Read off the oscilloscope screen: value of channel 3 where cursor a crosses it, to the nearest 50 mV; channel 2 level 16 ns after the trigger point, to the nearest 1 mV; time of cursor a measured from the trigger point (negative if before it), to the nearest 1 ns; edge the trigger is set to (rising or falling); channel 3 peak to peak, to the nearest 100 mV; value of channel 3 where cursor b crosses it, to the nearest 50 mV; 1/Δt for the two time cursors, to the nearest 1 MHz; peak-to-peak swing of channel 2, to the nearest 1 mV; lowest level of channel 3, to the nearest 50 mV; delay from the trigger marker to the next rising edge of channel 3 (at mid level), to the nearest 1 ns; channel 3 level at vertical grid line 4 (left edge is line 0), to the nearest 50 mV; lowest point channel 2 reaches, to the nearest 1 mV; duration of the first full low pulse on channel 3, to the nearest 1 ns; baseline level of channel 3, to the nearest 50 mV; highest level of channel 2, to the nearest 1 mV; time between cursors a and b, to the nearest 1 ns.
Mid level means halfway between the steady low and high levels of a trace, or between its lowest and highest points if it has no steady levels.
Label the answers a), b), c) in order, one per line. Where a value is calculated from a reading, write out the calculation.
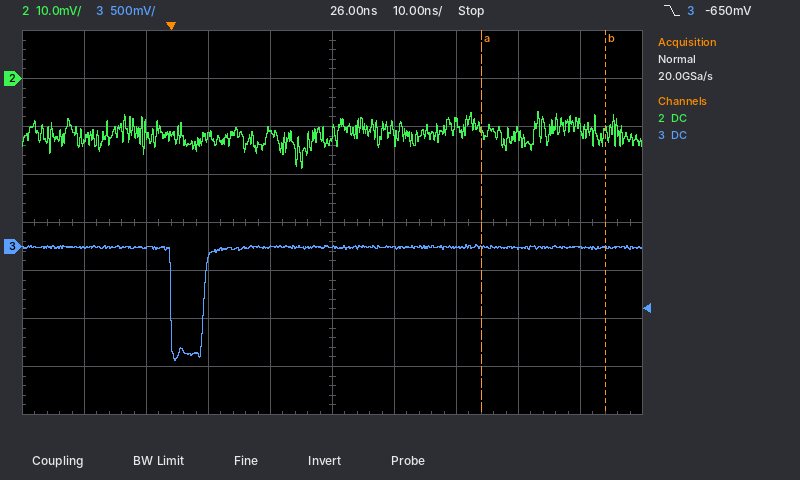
a) 0 mV
b) -11 mV
c) +50 ns
d) falling
e) 1.20 V
f) 0 mV
g) 1 / 20 ns ≈ 50 MHz
h) -7 mV − (-19 mV) = 12 mV
i) -1.20 V
j) 5 ns
k) 0 mV
l) -19 mV
m) 5 ns
n) 0 mV
o) -7 mV
p) 20 ns
